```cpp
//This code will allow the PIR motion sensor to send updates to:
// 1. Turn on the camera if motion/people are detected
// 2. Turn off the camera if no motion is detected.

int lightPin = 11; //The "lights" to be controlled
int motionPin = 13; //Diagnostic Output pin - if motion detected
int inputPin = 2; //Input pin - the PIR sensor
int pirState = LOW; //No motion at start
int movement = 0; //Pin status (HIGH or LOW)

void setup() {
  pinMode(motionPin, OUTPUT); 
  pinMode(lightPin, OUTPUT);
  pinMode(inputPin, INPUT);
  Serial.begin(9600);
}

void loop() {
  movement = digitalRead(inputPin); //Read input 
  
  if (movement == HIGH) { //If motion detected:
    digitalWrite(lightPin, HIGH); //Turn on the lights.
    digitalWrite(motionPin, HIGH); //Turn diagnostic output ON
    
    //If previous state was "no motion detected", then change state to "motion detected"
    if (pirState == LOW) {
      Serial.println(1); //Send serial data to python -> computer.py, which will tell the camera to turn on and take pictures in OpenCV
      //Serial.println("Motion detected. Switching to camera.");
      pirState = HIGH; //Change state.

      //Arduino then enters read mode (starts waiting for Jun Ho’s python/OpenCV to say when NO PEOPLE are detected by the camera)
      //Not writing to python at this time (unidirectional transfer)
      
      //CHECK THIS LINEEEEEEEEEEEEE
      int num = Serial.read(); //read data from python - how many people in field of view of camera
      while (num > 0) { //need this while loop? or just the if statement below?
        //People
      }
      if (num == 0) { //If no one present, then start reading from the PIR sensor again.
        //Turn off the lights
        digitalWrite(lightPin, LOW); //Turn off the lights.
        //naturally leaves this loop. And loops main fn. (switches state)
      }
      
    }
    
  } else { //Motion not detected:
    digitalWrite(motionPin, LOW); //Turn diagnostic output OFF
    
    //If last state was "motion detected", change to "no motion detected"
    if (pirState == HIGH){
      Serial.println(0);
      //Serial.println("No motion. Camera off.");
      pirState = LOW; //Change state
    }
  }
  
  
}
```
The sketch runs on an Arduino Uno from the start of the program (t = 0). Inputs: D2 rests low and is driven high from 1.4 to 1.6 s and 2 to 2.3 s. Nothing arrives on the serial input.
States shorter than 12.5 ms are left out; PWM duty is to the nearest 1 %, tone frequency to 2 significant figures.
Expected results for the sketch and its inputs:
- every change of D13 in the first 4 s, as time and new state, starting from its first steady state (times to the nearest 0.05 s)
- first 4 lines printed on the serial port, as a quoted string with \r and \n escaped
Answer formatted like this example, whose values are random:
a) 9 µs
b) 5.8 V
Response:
a) 0 s low; 1.4 s high; 1.6 s low; 2 s high; 2.3 s low
b) "1\r\n0\r\n1\r\n0\r\n"
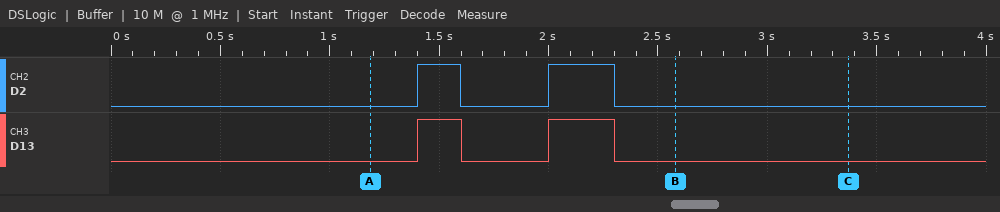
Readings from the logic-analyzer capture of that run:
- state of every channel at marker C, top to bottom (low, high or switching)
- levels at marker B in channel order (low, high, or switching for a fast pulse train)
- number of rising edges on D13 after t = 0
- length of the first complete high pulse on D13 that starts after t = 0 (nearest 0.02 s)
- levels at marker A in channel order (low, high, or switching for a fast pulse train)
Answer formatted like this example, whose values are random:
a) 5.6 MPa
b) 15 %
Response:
a) D2 low, D13 low
b) D2 low, D13 low
c) 2
d) 0.20 s
e) D2 low, D13 low
